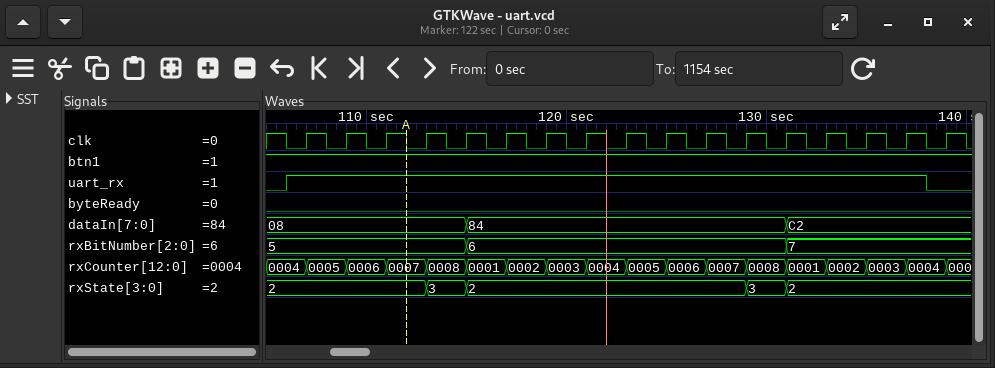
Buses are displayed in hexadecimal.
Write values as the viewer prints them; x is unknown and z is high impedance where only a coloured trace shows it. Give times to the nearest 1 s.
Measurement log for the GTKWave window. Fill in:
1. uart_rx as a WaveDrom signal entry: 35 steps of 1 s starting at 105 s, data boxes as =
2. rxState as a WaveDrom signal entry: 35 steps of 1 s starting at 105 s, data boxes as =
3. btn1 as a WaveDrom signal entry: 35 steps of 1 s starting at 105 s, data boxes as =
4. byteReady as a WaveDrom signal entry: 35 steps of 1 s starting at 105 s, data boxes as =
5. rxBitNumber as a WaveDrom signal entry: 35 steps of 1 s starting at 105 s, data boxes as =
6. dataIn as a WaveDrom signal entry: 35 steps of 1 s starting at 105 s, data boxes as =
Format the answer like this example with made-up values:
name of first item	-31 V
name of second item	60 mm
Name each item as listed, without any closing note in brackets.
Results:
uart_rx as a WaveDrom signal entry: 35 steps of 1 s starting at 105 s, data boxes as =	{name: 'uart_rx', wave: '01...............................0.'}
rxState as a WaveDrom signal entry: 35 steps of 1 s starting at 105 s, data boxes as =	{name: 'rxState', wave: '=.......=.=.............=.=........', data: '2 3 2 3 2'}
btn1 as a WaveDrom signal entry: 35 steps of 1 s starting at 105 s, data boxes as =	{name: 'btn1', wave: '1..................................'}
byteReady as a WaveDrom signal entry: 35 steps of 1 s starting at 105 s, data boxes as =	{name: 'byteReady', wave: '0..................................'}
rxBitNumber as a WaveDrom signal entry: 35 steps of 1 s starting at 105 s, data boxes as =	{name: 'rxBitNumber', wave: '=.........=...............=........', data: '5 6 7'}
dataIn as a WaveDrom signal entry: 35 steps of 1 s starting at 105 s, data boxes as =	{name: 'dataIn', wave: '=.........=...............=........', data: '08 84 C2'}
